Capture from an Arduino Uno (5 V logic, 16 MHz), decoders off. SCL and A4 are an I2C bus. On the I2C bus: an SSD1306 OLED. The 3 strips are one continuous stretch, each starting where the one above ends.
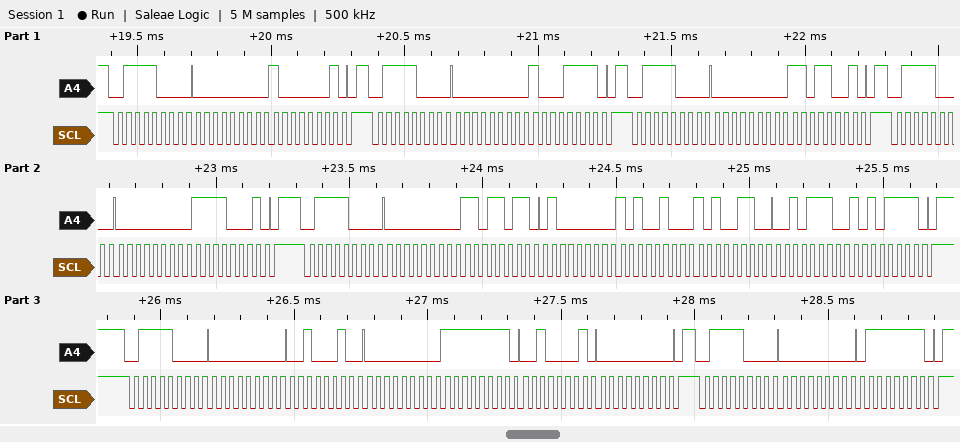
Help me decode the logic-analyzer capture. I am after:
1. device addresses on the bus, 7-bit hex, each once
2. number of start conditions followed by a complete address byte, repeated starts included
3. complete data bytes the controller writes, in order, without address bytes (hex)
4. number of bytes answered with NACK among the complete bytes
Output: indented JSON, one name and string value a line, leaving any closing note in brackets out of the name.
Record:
{
  "device addresses on the bus, 7-bit hex, each once": "0x3C",
  "number of start conditions followed by a complete address byte, repeated starts included": "7",
  "complete data bytes the controller writes, in order, without address bytes": "00 81 00 8F 00 D9 00 F1 00 DB 40 A4 A6 2E AF 00 22 00 FF 21 00 00 7F",
  "number of bytes answered with NACK among the complete bytes": "0"
}
